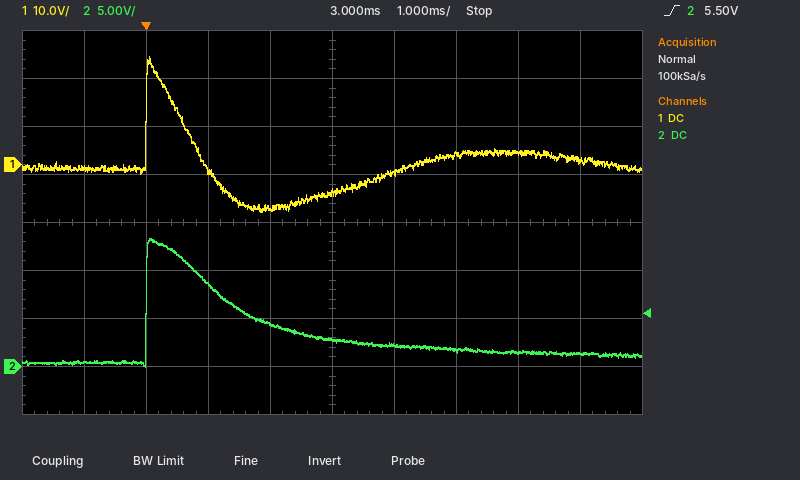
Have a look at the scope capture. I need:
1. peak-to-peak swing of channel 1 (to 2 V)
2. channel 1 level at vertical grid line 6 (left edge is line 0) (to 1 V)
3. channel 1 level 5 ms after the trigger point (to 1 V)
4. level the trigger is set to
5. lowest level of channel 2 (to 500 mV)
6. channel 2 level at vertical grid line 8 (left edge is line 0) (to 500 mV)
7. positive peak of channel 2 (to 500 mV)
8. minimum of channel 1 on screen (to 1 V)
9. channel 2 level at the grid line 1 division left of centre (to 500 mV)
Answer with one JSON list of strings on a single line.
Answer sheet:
["32 V", "-2 V", "2 V", "5.50 V", "0.0 V", "1.5 V", "13.5 V", "-10 V", "4.5 V"]
